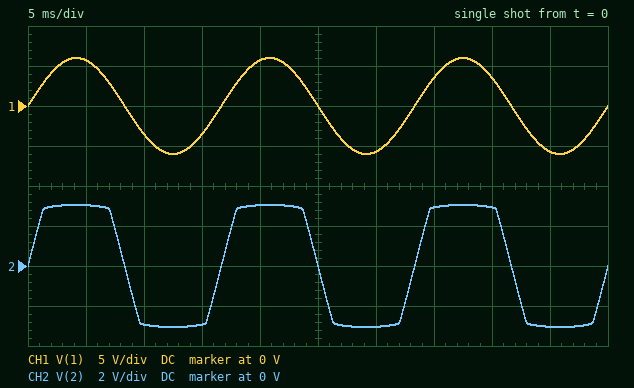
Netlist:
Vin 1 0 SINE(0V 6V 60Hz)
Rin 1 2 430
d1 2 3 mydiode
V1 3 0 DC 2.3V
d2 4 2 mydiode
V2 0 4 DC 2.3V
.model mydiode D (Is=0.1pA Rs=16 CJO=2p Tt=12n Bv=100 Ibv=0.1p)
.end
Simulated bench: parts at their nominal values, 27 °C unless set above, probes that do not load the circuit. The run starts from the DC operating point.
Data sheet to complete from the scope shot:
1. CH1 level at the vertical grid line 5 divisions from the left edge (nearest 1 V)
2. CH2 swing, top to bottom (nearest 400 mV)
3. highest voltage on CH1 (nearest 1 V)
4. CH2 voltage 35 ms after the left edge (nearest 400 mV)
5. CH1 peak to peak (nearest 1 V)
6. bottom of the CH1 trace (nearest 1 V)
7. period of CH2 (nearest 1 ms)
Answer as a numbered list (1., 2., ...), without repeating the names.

1. 0 V
2. 6.0 V
3. 6 V
4. 2.8 V
5. 12 V
6. -6 V
7. 17 ms
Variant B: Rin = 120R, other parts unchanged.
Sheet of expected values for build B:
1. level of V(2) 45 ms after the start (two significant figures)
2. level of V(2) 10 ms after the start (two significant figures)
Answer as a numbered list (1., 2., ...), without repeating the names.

1. -3.3 V
2. -3.0 V
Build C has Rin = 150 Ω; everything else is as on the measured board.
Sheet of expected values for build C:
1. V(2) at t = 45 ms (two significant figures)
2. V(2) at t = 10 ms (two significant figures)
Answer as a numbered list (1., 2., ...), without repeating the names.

1. -3.2 V
2. -3.0 V
